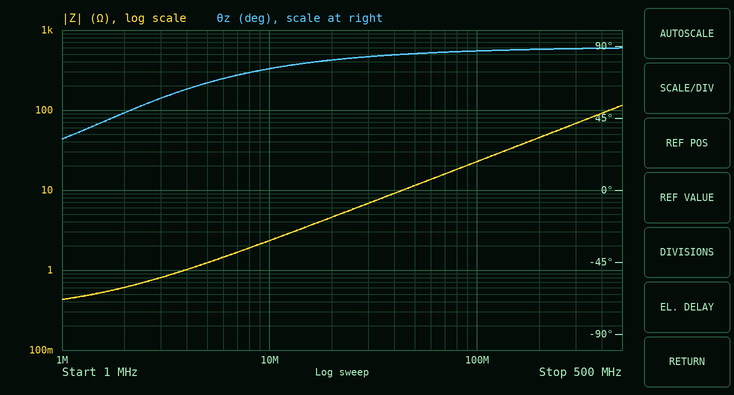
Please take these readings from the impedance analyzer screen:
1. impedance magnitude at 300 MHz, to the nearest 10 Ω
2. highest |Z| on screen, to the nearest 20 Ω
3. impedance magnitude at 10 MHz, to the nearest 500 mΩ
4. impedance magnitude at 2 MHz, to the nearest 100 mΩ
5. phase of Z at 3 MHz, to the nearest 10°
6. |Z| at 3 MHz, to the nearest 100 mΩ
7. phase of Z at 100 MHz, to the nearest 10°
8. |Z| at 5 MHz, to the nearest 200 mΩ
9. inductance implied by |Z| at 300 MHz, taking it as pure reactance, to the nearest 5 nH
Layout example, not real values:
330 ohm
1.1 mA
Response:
70 Ω
120 Ω
2.5 Ω
600 mΩ
60°
800 mΩ
90°
1.2 Ω
35 nH
